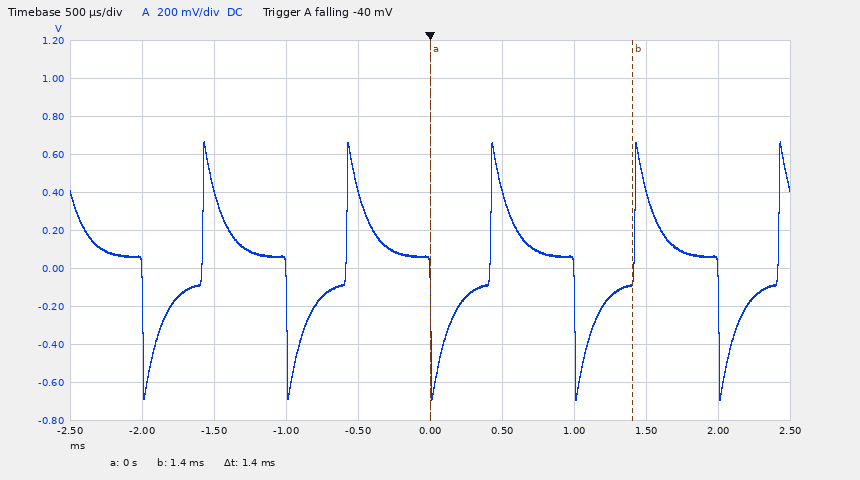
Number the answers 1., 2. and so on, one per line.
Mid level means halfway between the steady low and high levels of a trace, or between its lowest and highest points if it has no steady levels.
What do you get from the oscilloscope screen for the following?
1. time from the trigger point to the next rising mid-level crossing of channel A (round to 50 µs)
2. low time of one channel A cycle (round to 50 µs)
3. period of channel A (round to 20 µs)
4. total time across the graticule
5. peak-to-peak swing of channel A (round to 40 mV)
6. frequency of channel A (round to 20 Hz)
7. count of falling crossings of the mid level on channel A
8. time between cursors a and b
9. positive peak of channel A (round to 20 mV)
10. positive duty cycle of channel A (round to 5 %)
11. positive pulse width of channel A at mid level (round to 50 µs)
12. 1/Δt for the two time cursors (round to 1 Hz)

1. 400 µs
2. 400 µs
3. 1.00 ms
4. 5 ms
5. 1.36 V
6. 1.00 kHz
7. 5
8. 1.4 ms
9. 660 mV
10. 60 %
11. 600 µs
12. 714 Hz
